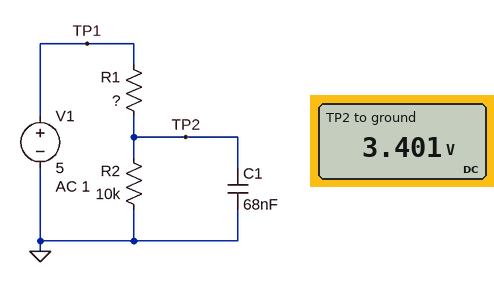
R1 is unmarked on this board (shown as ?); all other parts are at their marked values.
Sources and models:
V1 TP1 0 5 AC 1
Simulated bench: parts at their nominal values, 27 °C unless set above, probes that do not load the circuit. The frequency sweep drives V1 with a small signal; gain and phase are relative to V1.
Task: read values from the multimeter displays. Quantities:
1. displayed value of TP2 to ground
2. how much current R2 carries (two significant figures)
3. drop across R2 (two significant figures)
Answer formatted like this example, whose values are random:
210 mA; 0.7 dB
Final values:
3.401 V; 340 µA; 3.4 V
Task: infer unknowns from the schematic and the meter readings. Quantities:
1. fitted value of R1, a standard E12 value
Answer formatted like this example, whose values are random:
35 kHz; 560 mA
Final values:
4.7 kΩ
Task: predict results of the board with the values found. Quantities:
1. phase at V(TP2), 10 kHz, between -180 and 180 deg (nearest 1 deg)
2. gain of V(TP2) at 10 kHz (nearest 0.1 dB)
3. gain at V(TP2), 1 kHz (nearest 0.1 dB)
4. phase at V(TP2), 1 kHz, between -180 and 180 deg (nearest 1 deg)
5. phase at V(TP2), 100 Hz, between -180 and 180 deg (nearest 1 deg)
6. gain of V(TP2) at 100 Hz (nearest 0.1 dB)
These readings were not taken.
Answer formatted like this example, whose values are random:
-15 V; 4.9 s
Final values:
-86 deg; -26.1 dB; -7.9 dB; -54 deg; -8 deg; -3.4 dB
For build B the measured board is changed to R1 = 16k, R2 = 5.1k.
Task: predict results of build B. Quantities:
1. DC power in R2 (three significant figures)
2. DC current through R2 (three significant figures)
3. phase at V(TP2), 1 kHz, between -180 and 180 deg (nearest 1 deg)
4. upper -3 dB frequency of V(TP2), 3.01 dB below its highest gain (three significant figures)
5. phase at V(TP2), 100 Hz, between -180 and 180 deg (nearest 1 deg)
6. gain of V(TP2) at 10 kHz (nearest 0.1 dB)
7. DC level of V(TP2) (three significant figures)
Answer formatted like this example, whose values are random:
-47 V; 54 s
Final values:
286 µW; 237 µA; -59 deg; 605 Hz; -9 deg; -36.7 dB; 1.21 V
